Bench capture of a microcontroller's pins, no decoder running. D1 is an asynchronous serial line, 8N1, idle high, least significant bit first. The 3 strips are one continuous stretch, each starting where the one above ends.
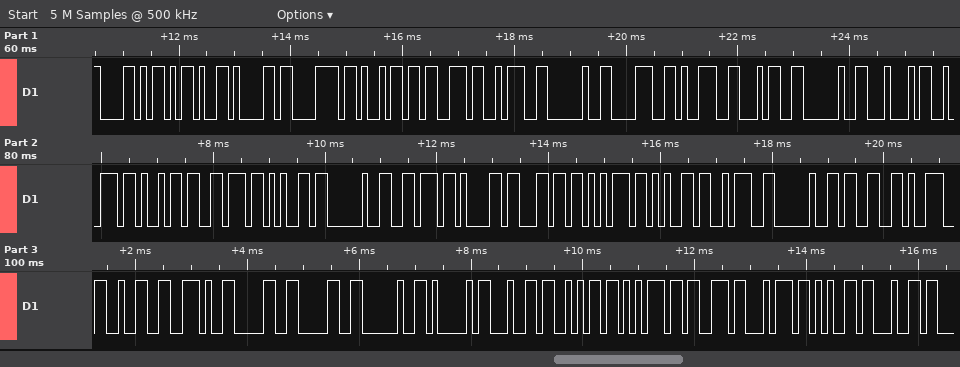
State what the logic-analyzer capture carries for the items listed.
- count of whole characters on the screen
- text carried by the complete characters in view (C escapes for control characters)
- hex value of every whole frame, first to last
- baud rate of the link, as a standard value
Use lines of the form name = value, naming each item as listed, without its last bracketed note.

count of whole characters on the screen = 40
text carried by the complete characters in view = "X-axis: 894 Drive value: 392.00 Adjusted"
hex value of every whole frame, first to last = 58 2D 61 78 69 73 3A 20 38 39 34 20 44 72 69 76 65 20 76 61 6C 75 65 3A 20 33 39 32 2E 30 30 20 41 64 6A 75 73 74 65 64
baud rate of the link, as a standard value = 9600 baud
